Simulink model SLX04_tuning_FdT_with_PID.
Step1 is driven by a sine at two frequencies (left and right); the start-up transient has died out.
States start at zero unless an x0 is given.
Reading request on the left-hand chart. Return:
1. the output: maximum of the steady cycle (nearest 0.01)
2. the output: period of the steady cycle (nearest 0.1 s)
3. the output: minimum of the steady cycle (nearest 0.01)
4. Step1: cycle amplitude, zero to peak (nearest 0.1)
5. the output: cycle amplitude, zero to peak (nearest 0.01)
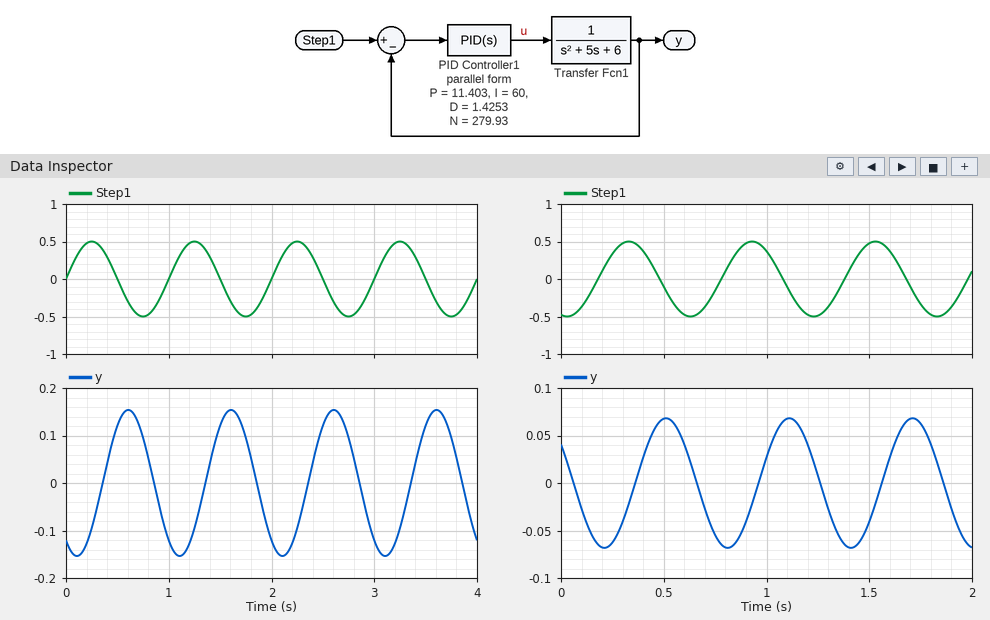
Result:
0.15
1.0 s
-0.15
0.5
0.15
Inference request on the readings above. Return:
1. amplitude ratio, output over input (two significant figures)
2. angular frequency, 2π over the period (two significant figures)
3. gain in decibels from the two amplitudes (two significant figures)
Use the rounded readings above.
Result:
0.30
6.3 rad/s
-10 dB
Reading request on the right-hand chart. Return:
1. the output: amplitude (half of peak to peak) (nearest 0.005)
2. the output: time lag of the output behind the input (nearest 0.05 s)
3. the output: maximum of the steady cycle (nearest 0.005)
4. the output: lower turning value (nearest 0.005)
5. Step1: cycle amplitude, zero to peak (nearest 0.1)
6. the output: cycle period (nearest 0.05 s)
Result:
0.070
0.20 s
0.070
-0.070
0.5
0.60 s
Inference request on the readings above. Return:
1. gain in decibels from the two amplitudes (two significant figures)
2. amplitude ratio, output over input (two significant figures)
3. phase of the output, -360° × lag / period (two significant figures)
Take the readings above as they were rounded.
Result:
-17 dB
0.14
-120°
